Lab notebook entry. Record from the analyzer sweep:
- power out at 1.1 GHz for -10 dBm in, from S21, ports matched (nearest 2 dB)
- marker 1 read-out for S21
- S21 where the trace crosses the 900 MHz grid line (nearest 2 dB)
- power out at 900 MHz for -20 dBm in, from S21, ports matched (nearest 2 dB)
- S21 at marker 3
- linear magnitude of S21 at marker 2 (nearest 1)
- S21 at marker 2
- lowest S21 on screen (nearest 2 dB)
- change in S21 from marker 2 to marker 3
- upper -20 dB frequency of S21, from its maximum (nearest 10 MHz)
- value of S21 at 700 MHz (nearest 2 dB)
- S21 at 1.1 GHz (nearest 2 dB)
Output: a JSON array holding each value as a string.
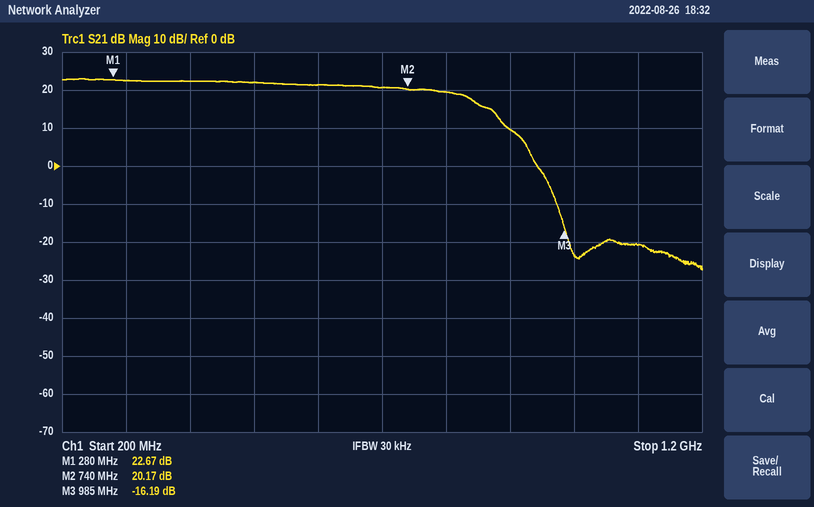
["-30 dBm", "22.67 dB", "10 dB", "-10 dBm", "-16.19 dB", "10", "20.17 dB", "-28 dB", "-36.36 dB", "930 MHz", "20 dB", "-20 dB"]
